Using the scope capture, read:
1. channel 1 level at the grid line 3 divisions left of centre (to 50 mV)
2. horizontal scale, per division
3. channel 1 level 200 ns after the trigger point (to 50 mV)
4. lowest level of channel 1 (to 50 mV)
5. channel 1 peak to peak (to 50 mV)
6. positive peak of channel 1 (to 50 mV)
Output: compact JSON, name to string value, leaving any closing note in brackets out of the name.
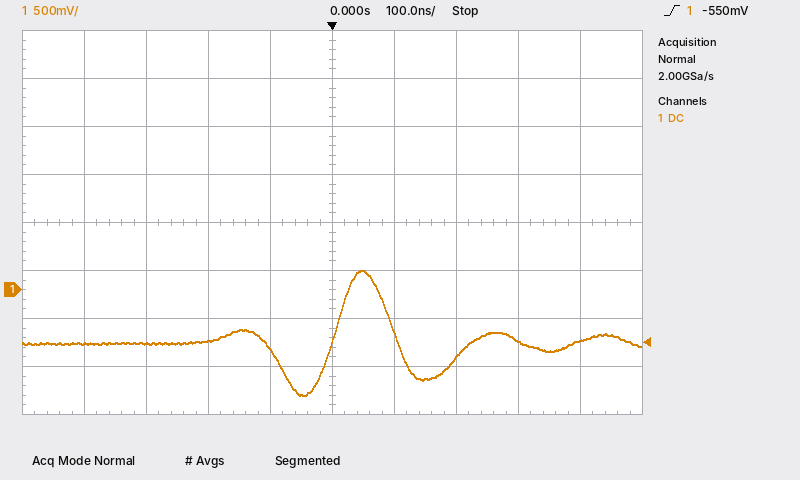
{"channel 1 level at the grid line 3 divisions left of centre": "-550 mV", "horizontal scale, per division": "100 ns", "channel 1 level 200 ns after the trigger point": "-700 mV", "lowest level of channel 1": "-1.10 V", "channel 1 peak to peak": "1.30 V", "positive peak of channel 1": "200 mV"}
